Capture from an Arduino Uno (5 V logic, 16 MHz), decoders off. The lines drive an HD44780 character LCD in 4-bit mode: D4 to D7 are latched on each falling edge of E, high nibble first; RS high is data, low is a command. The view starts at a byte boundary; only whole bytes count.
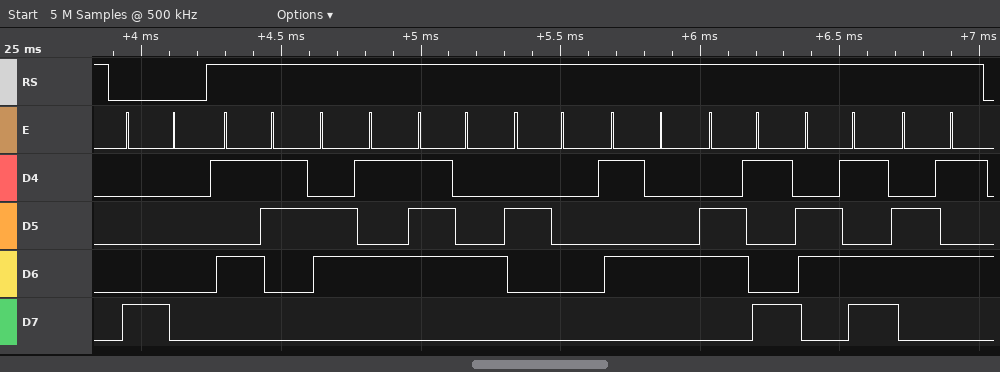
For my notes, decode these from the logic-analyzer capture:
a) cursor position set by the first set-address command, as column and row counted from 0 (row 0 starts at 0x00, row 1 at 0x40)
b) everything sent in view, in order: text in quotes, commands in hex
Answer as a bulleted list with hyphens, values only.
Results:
- column 0, row 0
- 0x80 "Set Time"
